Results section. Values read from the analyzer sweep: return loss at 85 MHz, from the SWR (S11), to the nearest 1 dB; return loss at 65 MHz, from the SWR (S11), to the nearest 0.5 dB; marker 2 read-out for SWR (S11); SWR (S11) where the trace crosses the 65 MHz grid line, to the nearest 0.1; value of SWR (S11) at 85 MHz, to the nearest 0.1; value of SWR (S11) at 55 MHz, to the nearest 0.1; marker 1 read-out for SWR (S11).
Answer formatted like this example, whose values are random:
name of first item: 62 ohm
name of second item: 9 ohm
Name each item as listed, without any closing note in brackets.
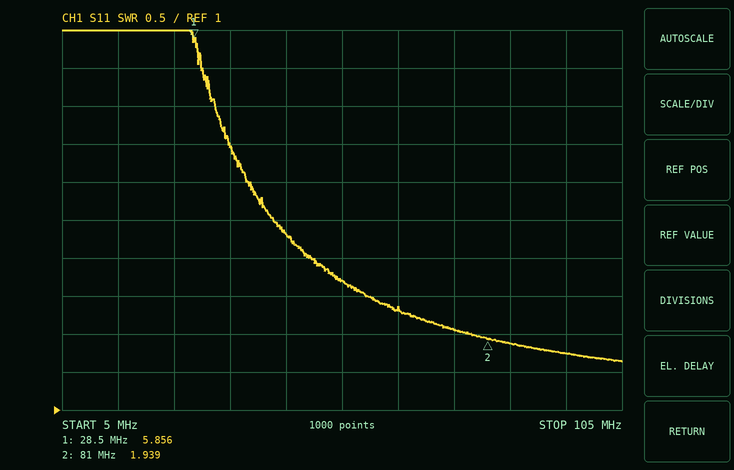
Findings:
return loss at 85 MHz, from the SWR (S11), to the nearest 1 dB: 10 dB
return loss at 65 MHz, from the SWR (S11), to the nearest 0.5 dB: 8.0 dB
marker 2 read-out for SWR: 1.939
SWR (S11) where the trace crosses the 65 MHz grid line, to the nearest 0.1: 2.3
value of SWR (S11) at 85 MHz, to the nearest 0.1: 1.9
value of SWR (S11) at 55 MHz, to the nearest 0.1: 2.7
marker 1 read-out for SWR: 5.856
